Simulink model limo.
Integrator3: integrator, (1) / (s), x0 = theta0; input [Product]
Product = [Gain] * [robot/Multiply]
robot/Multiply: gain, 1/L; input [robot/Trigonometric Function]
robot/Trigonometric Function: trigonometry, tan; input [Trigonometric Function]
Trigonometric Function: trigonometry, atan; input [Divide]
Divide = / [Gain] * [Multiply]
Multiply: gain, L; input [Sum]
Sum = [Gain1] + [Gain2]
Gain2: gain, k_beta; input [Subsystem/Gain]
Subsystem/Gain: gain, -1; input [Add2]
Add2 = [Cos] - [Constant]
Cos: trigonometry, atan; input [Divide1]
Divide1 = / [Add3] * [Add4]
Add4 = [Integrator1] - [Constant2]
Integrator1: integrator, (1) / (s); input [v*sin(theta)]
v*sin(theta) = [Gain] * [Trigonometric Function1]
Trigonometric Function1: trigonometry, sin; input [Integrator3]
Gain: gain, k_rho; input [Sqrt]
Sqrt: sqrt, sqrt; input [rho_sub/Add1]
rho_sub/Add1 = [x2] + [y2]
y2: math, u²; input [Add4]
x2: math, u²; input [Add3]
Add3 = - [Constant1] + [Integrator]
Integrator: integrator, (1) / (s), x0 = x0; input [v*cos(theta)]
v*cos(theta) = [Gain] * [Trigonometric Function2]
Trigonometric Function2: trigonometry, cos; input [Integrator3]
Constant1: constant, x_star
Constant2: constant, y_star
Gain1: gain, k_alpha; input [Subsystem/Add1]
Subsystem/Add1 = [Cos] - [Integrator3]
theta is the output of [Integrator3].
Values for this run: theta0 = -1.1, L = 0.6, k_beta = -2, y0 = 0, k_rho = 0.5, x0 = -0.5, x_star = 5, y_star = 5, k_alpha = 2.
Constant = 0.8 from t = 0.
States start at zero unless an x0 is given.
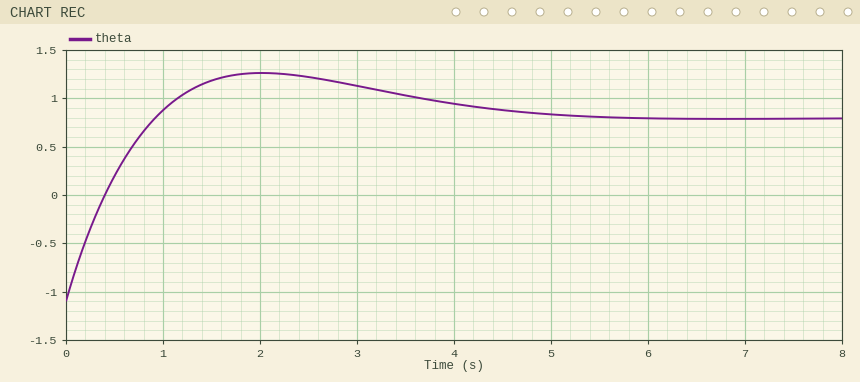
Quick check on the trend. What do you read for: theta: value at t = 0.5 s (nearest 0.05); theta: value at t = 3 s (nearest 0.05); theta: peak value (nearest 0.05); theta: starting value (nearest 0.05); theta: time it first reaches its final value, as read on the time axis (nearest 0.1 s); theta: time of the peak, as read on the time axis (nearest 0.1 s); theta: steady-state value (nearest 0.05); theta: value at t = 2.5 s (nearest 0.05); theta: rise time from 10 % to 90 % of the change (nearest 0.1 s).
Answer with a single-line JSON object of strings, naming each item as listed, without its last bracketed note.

{"theta: value at t = 0.5 s": "0.20", "theta: value at t = 3 s": "1.15", "theta: peak value": "1.25", "theta: starting value": "-1.10", "theta: time it first reaches its final value, as read on the time axis": "0.9 s", "theta: time of the peak, as read on the time axis": "2.0 s", "theta: steady-state value": "0.80", "theta: value at t = 2.5 s": "1.20", "theta: rise time from 10 % to 90 % of the change": "0.7 s"}
